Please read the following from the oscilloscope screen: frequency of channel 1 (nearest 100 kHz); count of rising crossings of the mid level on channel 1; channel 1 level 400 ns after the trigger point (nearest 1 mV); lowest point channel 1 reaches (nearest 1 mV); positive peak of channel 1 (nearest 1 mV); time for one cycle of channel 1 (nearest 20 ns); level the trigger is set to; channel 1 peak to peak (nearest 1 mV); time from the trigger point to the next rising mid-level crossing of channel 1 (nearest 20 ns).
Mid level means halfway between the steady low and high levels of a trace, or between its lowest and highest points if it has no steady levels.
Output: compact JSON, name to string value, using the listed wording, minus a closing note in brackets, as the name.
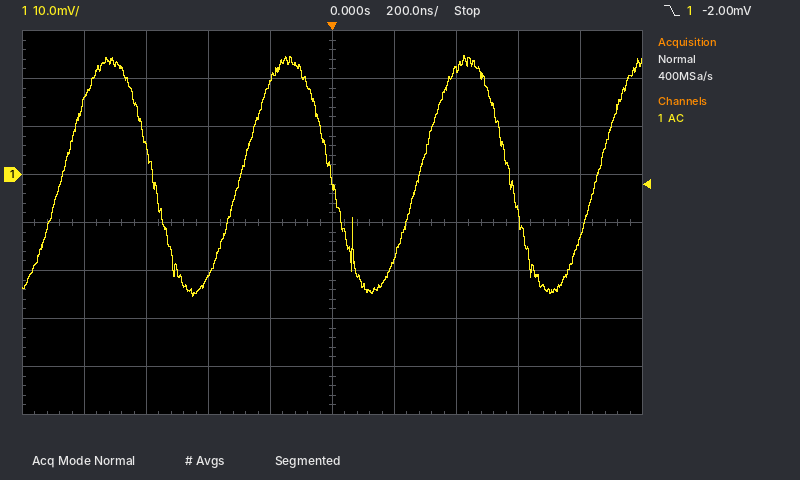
{"frequency of channel 1": "1.7 MHz", "count of rising crossings of the mid level on channel 1": "4", "channel 1 level 400 ns after the trigger point": "22 mV", "lowest point channel 1 reaches": "-25 mV", "positive peak of channel 1": "25 mV", "time for one cycle of channel 1": "580 ns", "level the trigger is set to": "-2.00 mV", "channel 1 peak to peak": "50 mV", "time from the trigger point to the next rising mid-level crossing of channel 1": "280 ns"}
